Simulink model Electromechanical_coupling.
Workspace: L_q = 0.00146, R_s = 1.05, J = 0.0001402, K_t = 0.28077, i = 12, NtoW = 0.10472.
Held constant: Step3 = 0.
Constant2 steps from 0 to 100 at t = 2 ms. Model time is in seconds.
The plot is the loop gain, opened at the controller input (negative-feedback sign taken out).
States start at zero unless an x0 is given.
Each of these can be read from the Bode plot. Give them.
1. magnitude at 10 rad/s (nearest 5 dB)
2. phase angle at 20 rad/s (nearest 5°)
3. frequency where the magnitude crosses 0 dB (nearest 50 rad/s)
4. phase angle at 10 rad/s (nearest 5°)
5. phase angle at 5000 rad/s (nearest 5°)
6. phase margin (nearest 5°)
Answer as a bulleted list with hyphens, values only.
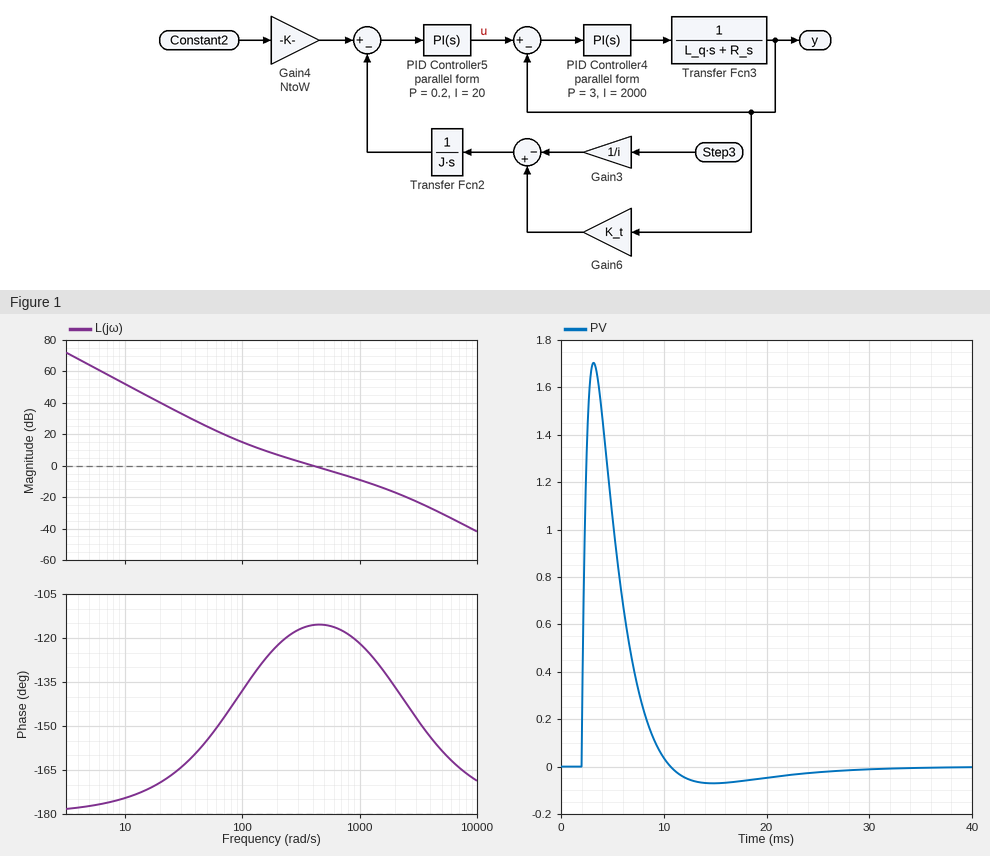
- 50 dB
- -170°
- 400 rad/s
- -175°
- -160°
- 65°
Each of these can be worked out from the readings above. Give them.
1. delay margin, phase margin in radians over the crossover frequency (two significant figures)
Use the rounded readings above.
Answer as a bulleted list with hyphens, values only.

- 0.0028 s
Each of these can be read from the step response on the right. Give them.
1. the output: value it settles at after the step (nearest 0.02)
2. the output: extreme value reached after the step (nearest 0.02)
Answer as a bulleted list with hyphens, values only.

- 0.00
- 1.70
